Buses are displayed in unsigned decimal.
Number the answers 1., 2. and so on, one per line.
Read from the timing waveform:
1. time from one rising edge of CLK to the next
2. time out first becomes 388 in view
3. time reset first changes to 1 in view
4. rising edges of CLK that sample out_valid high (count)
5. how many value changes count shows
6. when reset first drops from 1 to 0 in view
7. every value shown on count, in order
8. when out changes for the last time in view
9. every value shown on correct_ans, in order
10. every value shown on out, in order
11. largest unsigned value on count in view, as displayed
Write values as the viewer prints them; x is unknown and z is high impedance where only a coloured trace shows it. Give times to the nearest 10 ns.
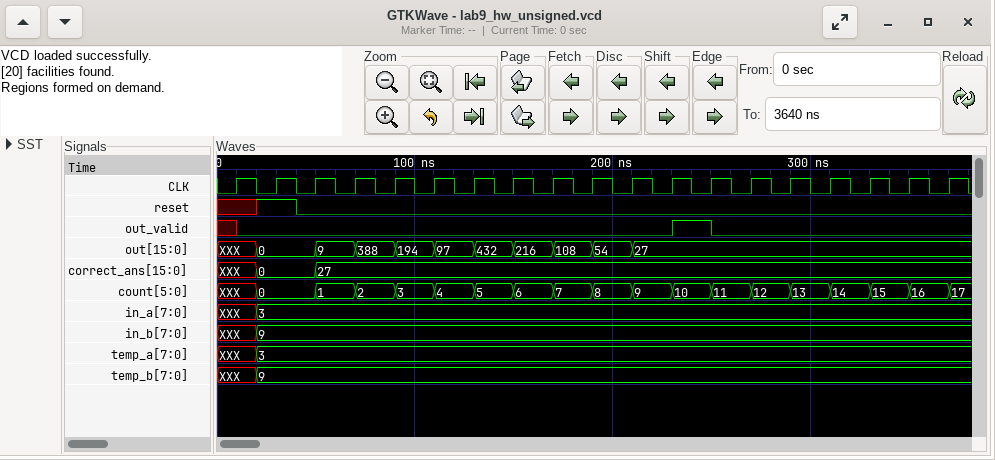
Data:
1. 20 ns
2. 70 ns
3. 20 ns
4. 1
5. 18
6. 40 ns
7. XXX, 0, 1, 2, 3, 4, 5, 6, 7, 8, 9, 10, 11, 12, 13, 14, 15, 16, 17
8. 210 ns
9. XXX, 0, 27
10. XXX, 0, 9, 388, 194, 97, 432, 216, 108, 54, 27
11. 17
